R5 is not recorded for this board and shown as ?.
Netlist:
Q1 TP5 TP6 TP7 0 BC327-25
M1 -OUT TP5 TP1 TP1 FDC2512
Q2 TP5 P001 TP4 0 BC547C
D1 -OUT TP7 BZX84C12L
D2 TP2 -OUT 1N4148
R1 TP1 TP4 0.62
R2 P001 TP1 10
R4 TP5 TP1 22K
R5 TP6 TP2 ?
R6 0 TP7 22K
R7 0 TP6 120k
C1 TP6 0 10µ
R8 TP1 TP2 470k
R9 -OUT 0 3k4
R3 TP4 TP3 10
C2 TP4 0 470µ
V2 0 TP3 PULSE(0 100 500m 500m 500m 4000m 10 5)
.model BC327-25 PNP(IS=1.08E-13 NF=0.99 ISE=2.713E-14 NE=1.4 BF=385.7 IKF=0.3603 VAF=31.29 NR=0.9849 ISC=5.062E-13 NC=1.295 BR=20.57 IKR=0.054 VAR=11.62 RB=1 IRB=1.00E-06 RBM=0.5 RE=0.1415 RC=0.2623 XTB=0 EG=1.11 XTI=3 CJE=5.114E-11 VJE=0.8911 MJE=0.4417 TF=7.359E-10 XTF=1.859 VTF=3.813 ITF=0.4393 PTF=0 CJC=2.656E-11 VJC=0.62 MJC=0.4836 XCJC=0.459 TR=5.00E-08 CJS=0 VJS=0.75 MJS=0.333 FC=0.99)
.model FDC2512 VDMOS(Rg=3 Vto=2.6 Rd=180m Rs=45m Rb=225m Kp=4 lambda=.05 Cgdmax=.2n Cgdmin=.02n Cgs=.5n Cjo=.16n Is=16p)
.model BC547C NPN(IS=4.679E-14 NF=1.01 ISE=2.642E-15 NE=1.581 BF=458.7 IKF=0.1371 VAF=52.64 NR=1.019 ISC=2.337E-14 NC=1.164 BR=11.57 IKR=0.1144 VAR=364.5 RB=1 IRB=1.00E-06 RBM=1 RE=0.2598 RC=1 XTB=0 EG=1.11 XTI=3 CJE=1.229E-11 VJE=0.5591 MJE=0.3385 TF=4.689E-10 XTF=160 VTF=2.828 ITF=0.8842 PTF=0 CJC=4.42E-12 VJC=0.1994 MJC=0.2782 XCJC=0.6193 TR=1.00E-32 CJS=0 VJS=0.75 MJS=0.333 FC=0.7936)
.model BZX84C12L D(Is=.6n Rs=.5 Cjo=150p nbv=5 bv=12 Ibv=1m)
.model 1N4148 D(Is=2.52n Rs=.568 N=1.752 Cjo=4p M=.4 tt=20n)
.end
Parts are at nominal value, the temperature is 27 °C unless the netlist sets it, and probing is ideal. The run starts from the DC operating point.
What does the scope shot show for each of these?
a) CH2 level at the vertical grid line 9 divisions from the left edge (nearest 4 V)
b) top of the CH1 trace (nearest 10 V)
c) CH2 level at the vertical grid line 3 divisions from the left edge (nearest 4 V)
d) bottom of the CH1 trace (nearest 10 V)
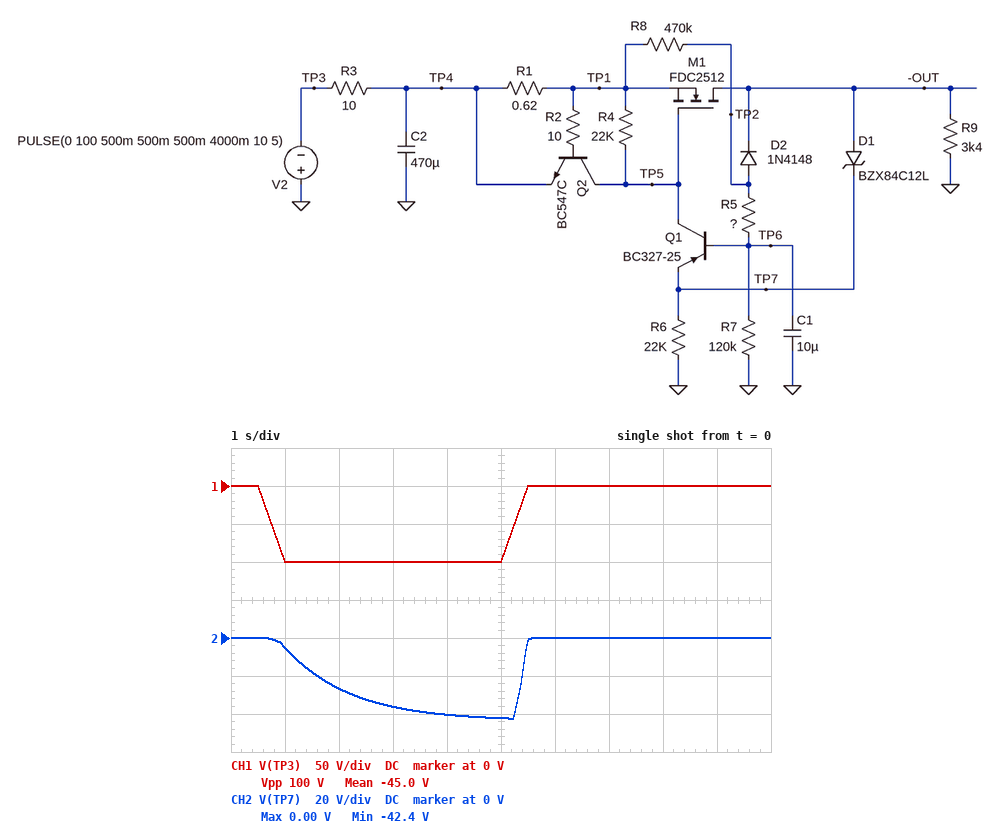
0 V
0 V
-36 V
-100 V
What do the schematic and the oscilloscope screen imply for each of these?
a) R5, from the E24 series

30 kΩ
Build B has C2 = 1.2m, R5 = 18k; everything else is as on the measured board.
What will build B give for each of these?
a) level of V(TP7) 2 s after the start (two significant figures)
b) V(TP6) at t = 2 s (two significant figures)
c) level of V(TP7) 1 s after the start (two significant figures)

-44 V
-45 V
-7.0 V
